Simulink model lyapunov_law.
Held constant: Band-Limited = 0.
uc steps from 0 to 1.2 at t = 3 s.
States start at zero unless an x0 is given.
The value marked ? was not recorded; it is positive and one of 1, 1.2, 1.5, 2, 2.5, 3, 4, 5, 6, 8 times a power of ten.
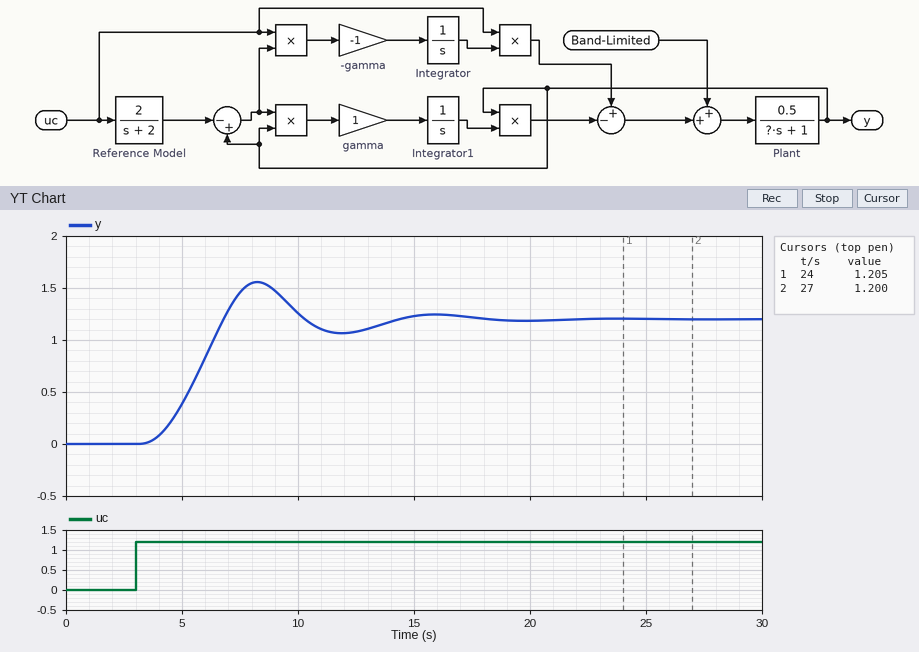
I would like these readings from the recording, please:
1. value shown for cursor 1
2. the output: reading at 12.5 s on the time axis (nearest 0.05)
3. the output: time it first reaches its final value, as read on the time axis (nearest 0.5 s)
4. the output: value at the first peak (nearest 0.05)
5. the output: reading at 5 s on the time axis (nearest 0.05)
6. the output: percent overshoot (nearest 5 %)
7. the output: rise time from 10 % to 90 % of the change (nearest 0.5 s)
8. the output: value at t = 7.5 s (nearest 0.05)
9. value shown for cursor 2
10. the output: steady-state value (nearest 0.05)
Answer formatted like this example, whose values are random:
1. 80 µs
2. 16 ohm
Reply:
1. 1.205
2. 1.10
3. 7.0 s
4. 1.55
5. 0.40
6. 30 %
7. 2.5 s
8. 1.45
9. 1.200
10. 1.20
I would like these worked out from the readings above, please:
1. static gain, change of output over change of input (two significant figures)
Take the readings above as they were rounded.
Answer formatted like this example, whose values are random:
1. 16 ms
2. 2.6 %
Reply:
1. 1.0
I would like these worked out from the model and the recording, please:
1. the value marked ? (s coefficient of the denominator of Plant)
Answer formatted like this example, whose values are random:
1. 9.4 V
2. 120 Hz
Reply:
1. 2
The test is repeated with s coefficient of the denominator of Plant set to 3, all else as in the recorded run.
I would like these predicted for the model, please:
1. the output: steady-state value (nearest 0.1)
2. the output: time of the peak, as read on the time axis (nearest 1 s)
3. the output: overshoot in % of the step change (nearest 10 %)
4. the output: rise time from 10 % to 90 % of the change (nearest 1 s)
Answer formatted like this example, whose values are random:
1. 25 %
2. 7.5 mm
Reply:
1. 1.2
2. 9 s
3. 40 %
4. 3 s
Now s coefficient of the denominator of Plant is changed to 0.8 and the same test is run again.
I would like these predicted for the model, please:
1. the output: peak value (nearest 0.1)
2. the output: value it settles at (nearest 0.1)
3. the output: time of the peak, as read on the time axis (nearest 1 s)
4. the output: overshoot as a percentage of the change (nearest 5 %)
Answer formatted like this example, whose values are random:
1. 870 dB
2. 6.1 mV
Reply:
1. 1.4
2. 1.2
3. 7 s
4. 15 %
